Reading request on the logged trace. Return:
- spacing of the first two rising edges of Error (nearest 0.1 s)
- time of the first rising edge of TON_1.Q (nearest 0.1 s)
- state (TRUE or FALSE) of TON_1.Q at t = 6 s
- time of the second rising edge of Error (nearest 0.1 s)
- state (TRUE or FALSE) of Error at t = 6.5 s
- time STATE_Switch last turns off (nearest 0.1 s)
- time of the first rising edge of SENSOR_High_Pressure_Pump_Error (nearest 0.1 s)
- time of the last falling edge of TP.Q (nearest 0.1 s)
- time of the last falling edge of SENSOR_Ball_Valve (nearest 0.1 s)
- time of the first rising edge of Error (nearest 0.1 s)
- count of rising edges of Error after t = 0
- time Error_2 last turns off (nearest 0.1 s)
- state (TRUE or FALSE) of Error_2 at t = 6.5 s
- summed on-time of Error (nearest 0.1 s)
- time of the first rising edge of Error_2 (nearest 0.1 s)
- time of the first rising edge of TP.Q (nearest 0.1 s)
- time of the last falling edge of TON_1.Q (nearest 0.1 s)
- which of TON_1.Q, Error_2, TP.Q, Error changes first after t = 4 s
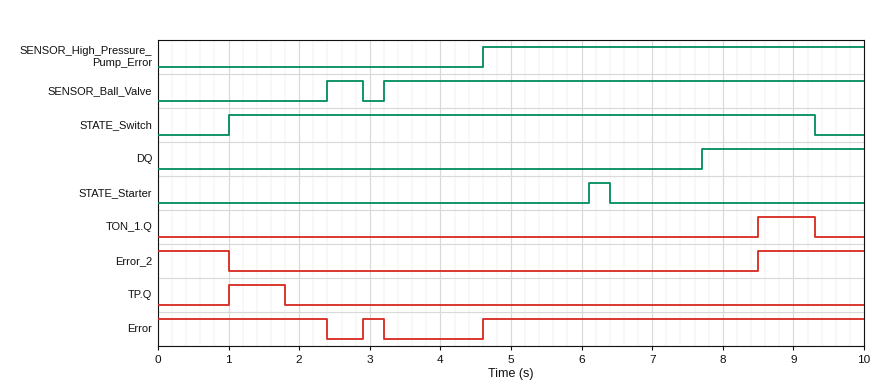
1.7 s
8.5 s
FALSE
4.6 s
TRUE
9.3 s
4.6 s
1.8 s
2.9 s
2.9 s
2
1.0 s
FALSE
8.1 s
8.5 s
1.0 s
9.3 s
Error
